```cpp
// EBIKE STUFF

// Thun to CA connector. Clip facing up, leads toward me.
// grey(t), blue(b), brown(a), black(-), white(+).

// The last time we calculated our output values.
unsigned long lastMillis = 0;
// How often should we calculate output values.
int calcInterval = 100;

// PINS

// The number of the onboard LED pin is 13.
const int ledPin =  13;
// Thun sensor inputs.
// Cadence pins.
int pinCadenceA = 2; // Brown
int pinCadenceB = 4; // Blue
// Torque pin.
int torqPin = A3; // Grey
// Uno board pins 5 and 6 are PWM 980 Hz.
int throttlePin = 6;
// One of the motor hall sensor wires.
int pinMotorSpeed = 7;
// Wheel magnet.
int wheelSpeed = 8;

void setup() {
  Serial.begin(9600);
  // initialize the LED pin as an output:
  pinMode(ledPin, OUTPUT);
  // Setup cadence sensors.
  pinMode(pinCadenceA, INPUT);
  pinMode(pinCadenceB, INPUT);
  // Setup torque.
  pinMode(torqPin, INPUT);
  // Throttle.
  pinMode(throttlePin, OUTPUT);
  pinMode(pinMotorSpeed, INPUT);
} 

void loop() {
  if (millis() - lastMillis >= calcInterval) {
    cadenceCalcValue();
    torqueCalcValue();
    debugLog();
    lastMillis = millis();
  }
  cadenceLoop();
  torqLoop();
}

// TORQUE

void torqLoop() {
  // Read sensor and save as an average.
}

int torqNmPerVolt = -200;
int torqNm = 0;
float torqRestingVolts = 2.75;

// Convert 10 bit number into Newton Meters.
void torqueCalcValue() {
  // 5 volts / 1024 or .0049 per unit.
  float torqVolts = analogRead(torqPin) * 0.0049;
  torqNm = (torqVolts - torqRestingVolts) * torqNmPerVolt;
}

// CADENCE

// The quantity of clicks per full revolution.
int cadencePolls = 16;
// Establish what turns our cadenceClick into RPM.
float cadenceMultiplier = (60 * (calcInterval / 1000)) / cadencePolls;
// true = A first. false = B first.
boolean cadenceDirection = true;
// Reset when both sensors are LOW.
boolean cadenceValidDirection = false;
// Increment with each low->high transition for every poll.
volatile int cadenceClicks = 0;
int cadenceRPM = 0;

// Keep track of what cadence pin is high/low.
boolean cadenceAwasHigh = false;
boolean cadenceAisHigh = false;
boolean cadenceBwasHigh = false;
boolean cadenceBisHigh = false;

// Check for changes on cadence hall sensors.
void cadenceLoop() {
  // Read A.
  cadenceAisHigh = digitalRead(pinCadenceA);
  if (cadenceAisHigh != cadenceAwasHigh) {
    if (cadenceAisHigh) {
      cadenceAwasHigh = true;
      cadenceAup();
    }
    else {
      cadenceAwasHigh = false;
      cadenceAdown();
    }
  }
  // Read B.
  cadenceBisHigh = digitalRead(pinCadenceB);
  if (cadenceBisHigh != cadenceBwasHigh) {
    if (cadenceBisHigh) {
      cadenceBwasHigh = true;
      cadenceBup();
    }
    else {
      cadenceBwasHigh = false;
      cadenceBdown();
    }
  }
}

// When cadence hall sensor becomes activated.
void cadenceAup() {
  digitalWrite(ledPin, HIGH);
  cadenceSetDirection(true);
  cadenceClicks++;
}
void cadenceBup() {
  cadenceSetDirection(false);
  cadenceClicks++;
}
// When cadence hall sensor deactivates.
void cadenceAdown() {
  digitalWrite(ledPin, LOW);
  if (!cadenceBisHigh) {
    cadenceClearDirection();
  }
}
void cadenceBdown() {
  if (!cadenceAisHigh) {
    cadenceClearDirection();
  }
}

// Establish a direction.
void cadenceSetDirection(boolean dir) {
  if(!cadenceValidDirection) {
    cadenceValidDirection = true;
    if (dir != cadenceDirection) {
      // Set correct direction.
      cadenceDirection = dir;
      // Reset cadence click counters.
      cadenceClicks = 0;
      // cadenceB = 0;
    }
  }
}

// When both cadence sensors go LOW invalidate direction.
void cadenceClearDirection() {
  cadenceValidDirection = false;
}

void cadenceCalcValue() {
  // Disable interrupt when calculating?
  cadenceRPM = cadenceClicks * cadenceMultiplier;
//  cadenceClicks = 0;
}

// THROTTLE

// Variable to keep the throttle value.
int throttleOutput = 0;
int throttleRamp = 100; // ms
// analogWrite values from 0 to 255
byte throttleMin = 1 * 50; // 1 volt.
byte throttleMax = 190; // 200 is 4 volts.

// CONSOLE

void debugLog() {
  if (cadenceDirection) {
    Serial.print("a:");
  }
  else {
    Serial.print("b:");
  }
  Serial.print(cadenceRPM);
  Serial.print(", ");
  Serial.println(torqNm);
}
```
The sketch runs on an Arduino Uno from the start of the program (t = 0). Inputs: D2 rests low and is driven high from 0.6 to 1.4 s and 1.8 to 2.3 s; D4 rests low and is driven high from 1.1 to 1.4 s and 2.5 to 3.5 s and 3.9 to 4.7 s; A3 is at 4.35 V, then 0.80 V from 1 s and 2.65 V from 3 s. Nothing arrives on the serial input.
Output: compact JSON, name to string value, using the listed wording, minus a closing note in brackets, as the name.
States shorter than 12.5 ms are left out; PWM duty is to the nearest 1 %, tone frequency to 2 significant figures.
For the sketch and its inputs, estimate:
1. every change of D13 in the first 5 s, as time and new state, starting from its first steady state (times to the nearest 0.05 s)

{"every change of D13 in the first 5 s, as time and new state, starting from its first steady state": "0 s low; 0.6 s high; 1.4 s low; 1.8 s high; 2.3 s low"}
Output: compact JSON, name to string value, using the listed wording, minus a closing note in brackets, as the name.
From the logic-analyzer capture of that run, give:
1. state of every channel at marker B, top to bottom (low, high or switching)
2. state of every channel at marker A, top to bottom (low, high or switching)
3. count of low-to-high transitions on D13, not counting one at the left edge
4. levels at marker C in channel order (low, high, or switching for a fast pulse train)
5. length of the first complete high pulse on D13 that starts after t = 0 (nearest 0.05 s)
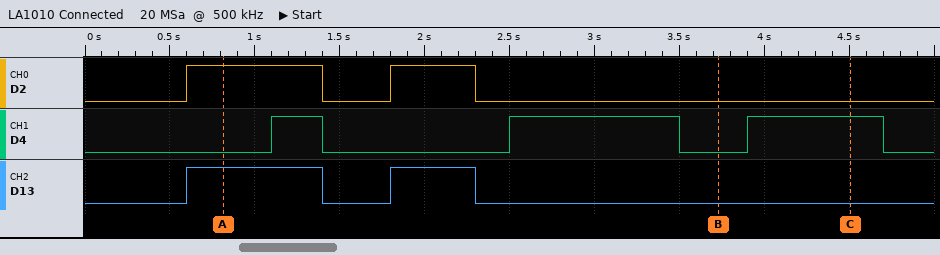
{"state of every channel at marker B, top to bottom": "D2 low, D4 low, D13 low", "state of every channel at marker A, top to bottom": "D2 high, D4 low, D13 high", "count of low-to-high transitions on D13, not counting one at the left edge": "2", "levels at marker C in channel order": "D2 low, D4 high, D13 low", "length of the first complete high pulse on D13 that starts after t = 0": "0.80 s"}
